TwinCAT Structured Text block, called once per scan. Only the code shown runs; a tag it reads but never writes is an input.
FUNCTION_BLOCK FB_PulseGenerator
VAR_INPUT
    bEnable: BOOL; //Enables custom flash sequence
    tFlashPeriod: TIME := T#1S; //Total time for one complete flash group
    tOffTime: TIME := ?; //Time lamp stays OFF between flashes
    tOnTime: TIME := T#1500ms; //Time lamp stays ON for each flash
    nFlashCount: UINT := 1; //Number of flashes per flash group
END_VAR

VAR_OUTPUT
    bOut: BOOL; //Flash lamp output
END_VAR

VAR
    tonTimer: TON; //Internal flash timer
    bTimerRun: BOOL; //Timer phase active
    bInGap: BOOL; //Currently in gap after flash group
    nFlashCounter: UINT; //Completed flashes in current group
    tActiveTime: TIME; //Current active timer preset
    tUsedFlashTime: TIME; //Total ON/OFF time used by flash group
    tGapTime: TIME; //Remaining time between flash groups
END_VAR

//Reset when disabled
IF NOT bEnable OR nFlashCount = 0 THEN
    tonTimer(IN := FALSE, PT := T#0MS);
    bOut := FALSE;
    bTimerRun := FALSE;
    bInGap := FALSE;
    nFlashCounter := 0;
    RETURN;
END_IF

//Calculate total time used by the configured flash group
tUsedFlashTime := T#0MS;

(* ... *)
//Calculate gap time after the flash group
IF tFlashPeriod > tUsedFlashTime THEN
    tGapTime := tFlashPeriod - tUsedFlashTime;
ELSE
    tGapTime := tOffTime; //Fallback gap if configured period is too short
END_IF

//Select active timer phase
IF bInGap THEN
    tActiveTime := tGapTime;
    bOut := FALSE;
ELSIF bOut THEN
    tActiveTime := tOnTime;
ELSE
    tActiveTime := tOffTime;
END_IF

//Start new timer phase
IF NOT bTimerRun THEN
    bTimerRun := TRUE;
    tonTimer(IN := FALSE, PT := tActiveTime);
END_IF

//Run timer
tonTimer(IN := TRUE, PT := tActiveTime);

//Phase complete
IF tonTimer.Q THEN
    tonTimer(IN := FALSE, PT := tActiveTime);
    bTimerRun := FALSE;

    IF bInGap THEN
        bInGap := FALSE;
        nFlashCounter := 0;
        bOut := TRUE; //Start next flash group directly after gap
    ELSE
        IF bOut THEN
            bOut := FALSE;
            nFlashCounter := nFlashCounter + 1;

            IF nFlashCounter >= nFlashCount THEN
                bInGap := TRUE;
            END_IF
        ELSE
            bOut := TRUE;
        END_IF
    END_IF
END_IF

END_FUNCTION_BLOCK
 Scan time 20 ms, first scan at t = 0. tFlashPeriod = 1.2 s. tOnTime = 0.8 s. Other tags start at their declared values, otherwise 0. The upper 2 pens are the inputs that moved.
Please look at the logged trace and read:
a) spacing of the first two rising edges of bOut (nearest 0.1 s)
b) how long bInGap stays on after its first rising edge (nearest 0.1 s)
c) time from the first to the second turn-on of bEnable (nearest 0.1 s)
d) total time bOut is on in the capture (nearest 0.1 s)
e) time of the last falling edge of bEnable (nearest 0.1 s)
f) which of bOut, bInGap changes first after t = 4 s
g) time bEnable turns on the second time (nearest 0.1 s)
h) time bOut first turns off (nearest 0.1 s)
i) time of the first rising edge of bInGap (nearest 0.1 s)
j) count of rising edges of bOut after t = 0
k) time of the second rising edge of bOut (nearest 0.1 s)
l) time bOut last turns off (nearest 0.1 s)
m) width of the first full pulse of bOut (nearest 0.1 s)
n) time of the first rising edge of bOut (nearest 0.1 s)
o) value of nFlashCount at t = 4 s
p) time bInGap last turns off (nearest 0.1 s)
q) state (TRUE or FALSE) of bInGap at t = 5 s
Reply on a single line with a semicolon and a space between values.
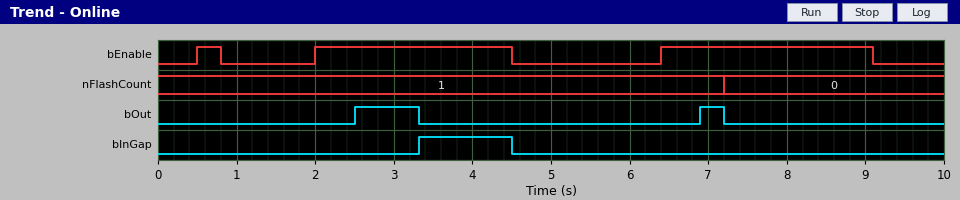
4.4 s; 1.2 s; 1.5 s; 1.1 s; 9.1 s; bInGap; 2.0 s; 3.3 s; 3.3 s; 2; 6.9 s; 7.2 s; 0.8 s; 2.5 s; 1; 4.5 s; FALSE
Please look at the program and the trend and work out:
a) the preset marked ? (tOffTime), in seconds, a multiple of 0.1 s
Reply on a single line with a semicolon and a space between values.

0.5 s
